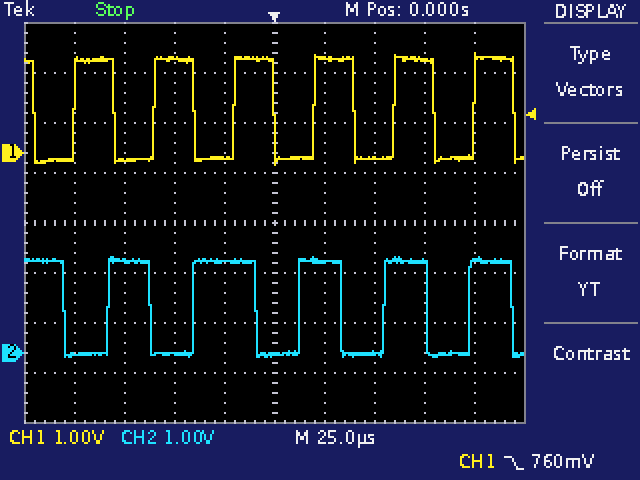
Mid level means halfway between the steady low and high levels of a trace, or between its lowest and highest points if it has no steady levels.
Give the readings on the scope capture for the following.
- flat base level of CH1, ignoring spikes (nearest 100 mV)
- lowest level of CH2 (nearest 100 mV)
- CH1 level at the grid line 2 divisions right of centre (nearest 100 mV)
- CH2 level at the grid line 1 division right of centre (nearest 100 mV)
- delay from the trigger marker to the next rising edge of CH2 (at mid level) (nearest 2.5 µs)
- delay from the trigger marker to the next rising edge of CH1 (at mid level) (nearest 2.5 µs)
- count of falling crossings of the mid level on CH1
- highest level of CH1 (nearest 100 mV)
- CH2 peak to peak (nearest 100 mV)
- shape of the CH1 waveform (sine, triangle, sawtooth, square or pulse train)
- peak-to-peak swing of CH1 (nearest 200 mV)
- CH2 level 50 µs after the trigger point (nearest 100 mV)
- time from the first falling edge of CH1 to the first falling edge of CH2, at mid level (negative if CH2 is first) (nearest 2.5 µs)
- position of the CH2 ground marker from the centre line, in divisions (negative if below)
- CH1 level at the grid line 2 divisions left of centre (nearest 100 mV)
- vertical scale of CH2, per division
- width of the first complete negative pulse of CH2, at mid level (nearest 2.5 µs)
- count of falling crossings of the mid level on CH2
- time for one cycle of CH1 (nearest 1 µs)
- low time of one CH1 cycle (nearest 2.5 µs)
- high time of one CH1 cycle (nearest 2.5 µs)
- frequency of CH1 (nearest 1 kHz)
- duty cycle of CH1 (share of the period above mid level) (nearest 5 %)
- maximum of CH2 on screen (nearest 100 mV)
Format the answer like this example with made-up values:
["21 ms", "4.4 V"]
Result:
["-100 mV", "-100 mV", "-100 mV", "1.8 V", "12.5 µs", "20.0 µs", "7", "2.0 V", "2.0 V", "square", "2.2 V", "0.0 V", "+15.0 µs", "-2.6 div", "1.9 V", "1 V", "22.5 µs", "6", "40 µs", "20.0 µs", "20.0 µs", "25 kHz", "50 %", "1.9 V"]
